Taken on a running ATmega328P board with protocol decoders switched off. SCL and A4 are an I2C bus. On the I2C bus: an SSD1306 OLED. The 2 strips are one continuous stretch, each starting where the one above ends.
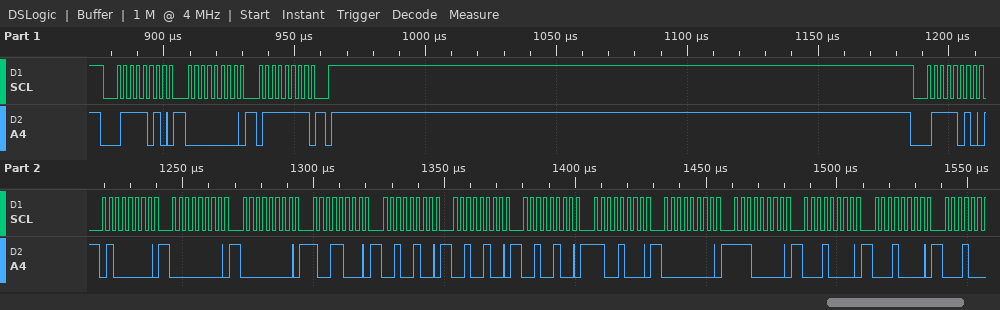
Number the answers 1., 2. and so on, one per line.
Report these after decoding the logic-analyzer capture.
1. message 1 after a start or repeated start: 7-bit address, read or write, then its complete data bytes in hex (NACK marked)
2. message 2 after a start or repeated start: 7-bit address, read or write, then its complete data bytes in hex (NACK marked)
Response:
1. 0x3D write: 00 7F
2. 0x3D write: 40 00 00 98 24 24 24 C8 00 E0 10 10
